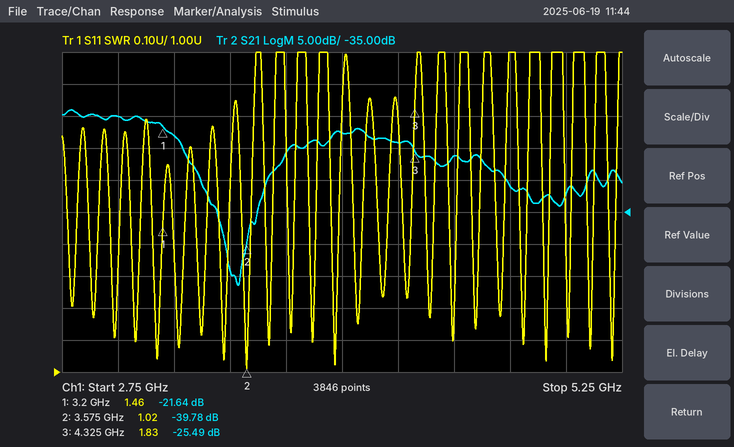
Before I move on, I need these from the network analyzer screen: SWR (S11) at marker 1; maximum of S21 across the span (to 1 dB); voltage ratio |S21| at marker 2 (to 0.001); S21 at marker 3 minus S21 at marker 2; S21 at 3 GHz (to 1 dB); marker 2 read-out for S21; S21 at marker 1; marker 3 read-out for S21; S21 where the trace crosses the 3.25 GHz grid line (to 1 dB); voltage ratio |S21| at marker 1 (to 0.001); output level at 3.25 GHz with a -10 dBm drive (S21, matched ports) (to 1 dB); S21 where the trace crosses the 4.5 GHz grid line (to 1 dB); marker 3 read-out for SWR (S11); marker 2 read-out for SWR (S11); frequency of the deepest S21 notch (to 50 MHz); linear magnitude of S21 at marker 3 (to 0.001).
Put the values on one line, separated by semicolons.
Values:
1.46; -19 dB; 0.010; 14.29 dB; -20 dB; -39.78 dB; -21.64 dB; -25.49 dB; -23 dB; 0.083; -33 dBm; -26 dB; 1.83; 1.02; 3.55 GHz; 0.053
